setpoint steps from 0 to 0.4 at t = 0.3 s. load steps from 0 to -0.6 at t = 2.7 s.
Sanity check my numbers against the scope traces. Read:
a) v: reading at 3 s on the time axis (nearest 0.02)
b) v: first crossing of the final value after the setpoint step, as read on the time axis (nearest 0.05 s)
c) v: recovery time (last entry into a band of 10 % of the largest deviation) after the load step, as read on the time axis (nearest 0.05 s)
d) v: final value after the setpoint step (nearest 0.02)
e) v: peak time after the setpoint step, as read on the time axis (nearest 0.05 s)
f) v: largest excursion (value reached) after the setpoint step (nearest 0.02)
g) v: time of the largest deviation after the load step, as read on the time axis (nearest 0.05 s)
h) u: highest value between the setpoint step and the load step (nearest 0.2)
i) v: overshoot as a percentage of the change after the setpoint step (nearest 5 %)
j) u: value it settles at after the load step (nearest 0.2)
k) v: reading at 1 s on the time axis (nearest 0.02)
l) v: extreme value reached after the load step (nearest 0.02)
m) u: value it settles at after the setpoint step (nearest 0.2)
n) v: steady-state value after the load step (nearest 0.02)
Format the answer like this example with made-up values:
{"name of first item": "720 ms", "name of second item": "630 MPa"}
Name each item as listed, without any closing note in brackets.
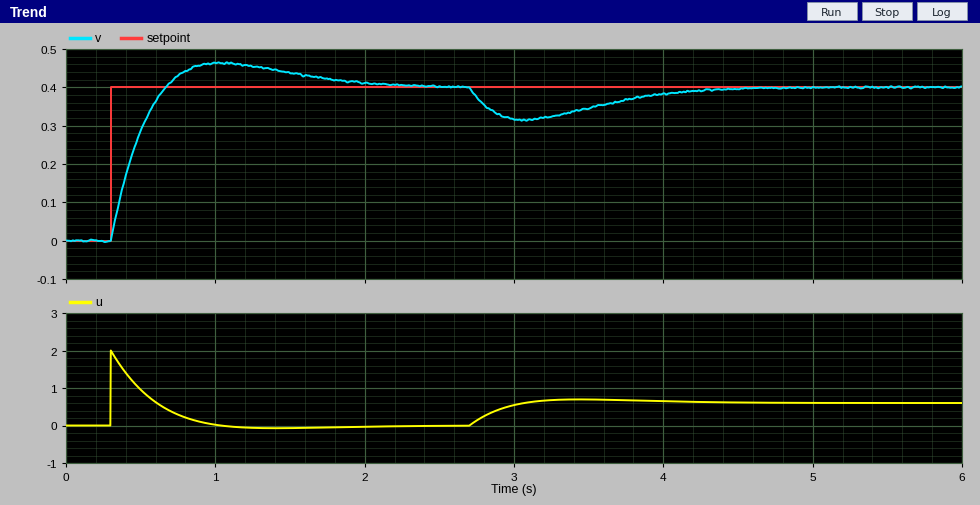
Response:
{"v: reading at 3 s on the time axis": "0.32", "v: first crossing of the final value after the setpoint step, as read on the time axis": "0.65 s", "v: recovery time (last entry into a band of 10 % of the largest deviation) after the load step, as read on the time axis": "4.25 s", "v: final value after the setpoint step": "0.40", "v: peak time after the setpoint step, as read on the time axis": "1.05 s", "v: largest excursion (value reached) after the setpoint step": "0.46", "v: time of the largest deviation after the load step, as read on the time axis": "3.05 s", "u: highest value between the setpoint step and the load step": "2.0", "v: overshoot as a percentage of the change after the setpoint step": "15 %", "u: value it settles at after the load step": "0.6", "v: reading at 1 s on the time axis": "0.46", "v: extreme value reached after the load step": "0.32", "u: value it settles at after the setpoint step": "0.0", "v: steady-state value after the load step": "0.40"}
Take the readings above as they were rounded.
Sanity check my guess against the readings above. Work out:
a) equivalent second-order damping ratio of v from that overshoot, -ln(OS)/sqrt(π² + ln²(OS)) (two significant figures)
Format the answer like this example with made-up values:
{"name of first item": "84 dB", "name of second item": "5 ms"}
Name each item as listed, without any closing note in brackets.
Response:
{"equivalent second-order damping ratio of v from that overshoot, -ln(OS)/sqrt(π² + ln²(OS))": "0.52"}
